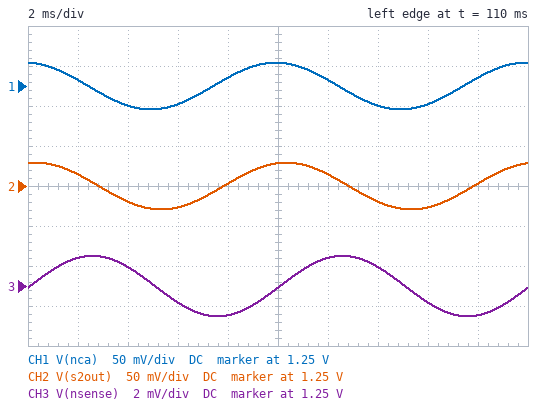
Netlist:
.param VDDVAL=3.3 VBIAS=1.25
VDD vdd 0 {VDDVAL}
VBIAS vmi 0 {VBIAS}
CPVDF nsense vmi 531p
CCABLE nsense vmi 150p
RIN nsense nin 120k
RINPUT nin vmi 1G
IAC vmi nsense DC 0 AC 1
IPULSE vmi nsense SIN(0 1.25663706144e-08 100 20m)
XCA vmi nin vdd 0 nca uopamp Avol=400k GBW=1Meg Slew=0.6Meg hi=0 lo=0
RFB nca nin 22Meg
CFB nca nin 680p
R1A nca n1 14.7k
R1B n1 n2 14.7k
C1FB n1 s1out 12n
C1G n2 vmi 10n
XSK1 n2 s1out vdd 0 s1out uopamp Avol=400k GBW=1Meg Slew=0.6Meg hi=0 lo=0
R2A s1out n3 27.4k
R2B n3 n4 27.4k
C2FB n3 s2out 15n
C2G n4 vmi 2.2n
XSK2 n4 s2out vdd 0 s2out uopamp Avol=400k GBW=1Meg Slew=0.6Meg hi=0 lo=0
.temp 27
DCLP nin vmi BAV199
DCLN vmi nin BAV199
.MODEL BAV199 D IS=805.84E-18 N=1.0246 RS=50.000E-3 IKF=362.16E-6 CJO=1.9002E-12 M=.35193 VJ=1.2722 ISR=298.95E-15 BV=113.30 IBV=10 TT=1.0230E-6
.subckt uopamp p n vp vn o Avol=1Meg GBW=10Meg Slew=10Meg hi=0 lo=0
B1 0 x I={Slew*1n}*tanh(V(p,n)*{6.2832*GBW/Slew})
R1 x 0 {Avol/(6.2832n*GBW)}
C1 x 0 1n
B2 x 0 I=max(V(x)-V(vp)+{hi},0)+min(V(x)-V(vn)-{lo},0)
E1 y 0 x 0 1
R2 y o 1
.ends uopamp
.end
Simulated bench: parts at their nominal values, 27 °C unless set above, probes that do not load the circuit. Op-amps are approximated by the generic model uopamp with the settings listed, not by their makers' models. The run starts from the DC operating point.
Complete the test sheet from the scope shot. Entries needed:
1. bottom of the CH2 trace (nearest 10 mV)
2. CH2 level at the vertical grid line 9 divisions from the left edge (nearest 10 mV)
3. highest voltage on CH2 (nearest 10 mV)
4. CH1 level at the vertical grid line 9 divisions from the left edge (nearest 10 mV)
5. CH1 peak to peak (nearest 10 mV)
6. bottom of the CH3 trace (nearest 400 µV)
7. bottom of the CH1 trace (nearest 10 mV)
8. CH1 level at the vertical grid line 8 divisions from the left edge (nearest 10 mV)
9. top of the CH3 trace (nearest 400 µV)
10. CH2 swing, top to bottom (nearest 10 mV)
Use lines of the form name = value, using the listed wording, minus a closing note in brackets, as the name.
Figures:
bottom of the CH2 trace = 1.22 V
CH2 level at the vertical grid line 9 divisions from the left edge = 1.25 V
highest voltage on CH2 = 1.28 V
CH1 level at the vertical grid line 9 divisions from the left edge = 1.26 V
CH1 peak to peak = 60 mV
bottom of the CH3 trace = 1.2484 V
bottom of the CH1 trace = 1.22 V
CH1 level at the vertical grid line 8 divisions from the left edge = 1.23 V
top of the CH3 trace = 1.2516 V
CH2 swing, top to bottom = 60 mV
